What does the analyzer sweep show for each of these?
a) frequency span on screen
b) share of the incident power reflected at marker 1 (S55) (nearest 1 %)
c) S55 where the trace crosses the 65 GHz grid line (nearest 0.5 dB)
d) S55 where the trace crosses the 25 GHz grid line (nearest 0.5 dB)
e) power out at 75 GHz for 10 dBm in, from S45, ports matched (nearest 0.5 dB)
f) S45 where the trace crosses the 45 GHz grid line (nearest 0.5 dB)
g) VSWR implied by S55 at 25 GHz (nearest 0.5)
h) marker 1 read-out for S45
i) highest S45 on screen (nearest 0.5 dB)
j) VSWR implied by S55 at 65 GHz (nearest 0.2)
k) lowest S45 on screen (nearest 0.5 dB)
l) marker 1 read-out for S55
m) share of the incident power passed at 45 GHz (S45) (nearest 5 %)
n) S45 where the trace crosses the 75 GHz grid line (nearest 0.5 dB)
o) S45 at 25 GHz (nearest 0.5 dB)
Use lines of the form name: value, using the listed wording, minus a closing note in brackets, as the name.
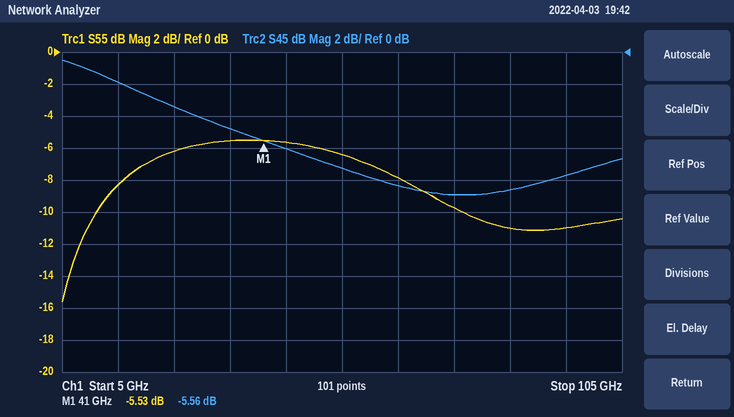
frequency span on screen: 100 GHz
share of the incident power reflected at marker 1 (S55): 28 %
S55 where the trace crosses the 65 GHz grid line: -8.0 dB
S55 where the trace crosses the 25 GHz grid line: -6.0 dB
power out at 75 GHz for 10 dBm in, from S45, ports matched: 1.0 dBm
S45 where the trace crosses the 45 GHz grid line: -6.0 dB
VSWR implied by S55 at 25 GHz: 3.0
marker 1 read-out for S45: -5.56 dB
highest S45 on screen: -0.5 dB
VSWR implied by S55 at 65 GHz: 2.4
lowest S45 on screen: -9.0 dB
marker 1 read-out for S55: -5.53 dB
share of the incident power passed at 45 GHz (S45): 25 %
S45 where the trace crosses the 75 GHz grid line: -9.0 dB
S45 at 25 GHz: -3.5 dB
